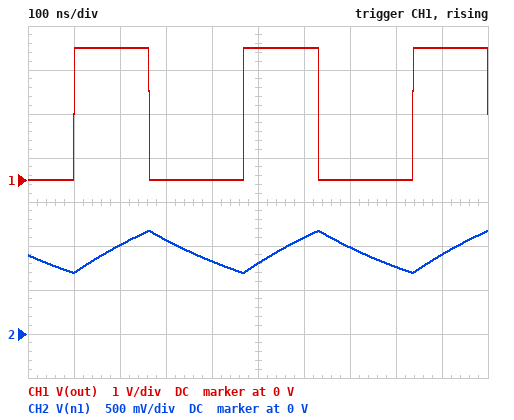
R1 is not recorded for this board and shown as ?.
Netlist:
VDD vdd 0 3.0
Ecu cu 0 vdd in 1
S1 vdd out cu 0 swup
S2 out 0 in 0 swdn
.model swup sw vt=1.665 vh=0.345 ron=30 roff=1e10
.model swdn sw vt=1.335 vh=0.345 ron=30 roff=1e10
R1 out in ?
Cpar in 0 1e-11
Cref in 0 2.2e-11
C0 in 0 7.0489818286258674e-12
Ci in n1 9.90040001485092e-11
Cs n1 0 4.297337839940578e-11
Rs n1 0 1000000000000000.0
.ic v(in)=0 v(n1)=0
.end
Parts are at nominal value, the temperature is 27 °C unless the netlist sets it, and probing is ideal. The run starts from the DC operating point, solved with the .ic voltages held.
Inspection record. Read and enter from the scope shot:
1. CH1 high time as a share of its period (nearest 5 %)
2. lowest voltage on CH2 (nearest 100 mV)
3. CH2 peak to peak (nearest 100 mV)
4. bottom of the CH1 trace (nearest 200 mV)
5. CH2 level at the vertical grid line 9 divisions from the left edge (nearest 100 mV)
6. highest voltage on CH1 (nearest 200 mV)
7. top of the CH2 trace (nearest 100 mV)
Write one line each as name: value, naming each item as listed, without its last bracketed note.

CH1 high time as a share of its period: 45 %
lowest voltage on CH2: 700 mV
CH2 peak to peak: 500 mV
bottom of the CH1 trace: 0 V
CH2 level at the vertical grid line 9 divisions from the left edge: 900 mV
highest voltage on CH1: 3.0 V
top of the CH2 trace: 1.2 V
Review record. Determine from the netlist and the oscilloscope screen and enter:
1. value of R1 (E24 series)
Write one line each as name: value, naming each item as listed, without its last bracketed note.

value of R1: 5.6 kΩ
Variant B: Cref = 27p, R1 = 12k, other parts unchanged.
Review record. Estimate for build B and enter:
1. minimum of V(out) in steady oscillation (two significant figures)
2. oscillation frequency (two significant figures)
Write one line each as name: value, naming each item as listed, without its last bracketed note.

minimum of V(out) in steady oscillation: 2.5 mV
oscillation frequency: 1.2 MHz
